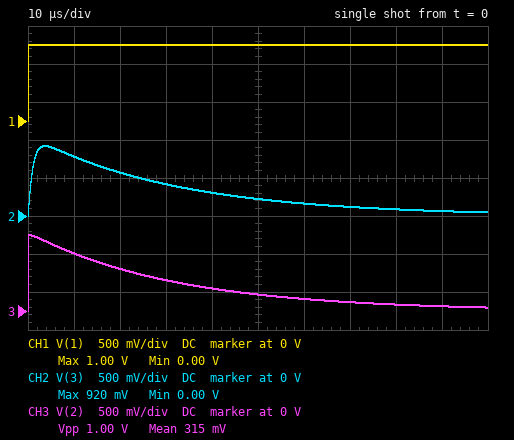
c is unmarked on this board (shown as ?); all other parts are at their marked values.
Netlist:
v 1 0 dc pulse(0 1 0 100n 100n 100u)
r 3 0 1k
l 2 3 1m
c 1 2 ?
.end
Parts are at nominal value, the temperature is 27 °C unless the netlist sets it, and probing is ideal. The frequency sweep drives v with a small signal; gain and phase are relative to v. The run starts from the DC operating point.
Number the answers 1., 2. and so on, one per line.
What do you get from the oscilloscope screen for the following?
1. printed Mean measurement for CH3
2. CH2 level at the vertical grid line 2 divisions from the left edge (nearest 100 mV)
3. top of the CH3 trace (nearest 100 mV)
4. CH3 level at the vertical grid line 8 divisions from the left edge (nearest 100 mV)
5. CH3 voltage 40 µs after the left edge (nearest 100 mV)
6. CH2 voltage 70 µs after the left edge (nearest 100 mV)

1. 315 mV
2. 600 mV
3. 1.0 V
4. 100 mV
5. 300 mV
6. 100 mV
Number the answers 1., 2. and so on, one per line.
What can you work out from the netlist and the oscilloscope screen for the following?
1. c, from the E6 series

1. 33 nF
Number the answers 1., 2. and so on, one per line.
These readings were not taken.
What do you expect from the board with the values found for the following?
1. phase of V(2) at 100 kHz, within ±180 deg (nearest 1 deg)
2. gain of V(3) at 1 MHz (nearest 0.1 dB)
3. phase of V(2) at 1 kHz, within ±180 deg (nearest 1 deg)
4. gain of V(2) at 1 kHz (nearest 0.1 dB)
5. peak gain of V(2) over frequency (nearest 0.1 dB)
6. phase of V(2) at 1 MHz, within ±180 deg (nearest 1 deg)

1. 2 deg
2. -16.1 dB
3. 79 deg
4. -13.8 dB
5. 0.2 dB
6. 0 deg
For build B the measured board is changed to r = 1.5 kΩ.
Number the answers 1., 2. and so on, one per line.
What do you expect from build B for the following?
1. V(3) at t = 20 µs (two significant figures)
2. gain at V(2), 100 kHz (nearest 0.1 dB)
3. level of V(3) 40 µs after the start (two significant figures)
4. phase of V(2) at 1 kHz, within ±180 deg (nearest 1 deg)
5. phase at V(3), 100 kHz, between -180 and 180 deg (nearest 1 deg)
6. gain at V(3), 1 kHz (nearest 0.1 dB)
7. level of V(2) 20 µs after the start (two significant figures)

1. 680 mV
2. 0.1 dB
3. 450 mV
4. 73 deg
5. -21 deg
6. -10.5 dB
7. 670 mV
